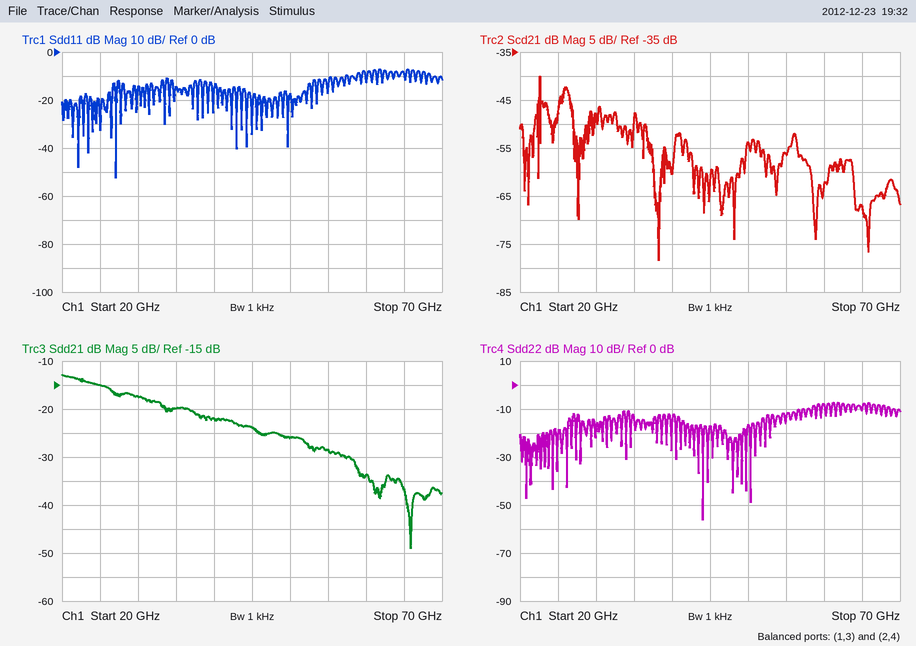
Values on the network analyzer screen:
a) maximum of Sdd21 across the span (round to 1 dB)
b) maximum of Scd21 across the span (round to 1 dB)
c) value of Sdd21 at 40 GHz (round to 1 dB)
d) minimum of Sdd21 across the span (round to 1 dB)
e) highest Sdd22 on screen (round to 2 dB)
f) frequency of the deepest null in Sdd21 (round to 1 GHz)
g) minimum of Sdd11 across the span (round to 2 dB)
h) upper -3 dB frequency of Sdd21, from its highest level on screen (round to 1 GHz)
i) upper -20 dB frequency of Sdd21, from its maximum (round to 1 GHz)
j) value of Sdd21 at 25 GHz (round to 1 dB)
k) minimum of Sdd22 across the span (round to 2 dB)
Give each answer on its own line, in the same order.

-13 dB
-40 dB
-22 dB
-49 dB
-8 dB
66 GHz
-52 dB
26 GHz
59 GHz
-15 dB
-56 dB
